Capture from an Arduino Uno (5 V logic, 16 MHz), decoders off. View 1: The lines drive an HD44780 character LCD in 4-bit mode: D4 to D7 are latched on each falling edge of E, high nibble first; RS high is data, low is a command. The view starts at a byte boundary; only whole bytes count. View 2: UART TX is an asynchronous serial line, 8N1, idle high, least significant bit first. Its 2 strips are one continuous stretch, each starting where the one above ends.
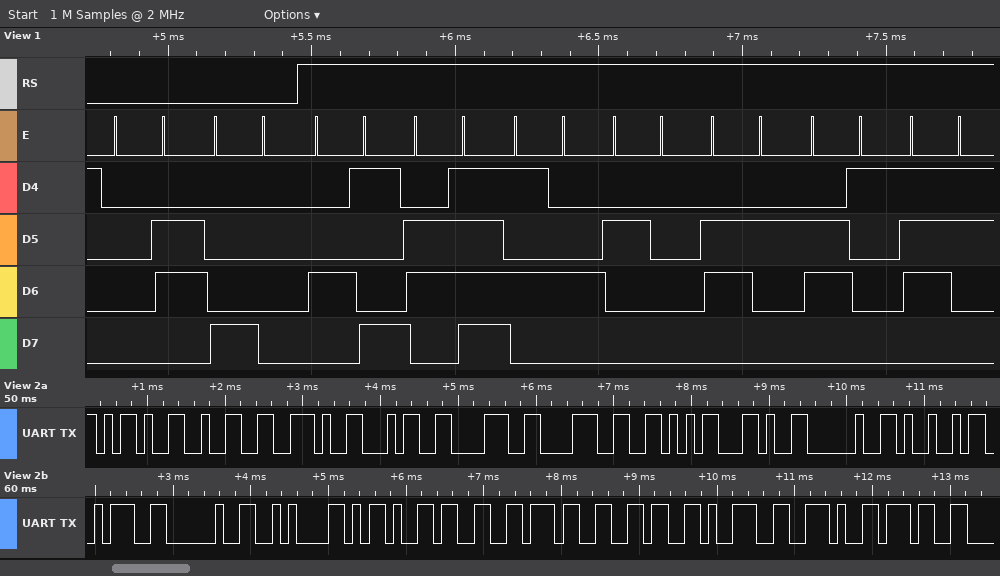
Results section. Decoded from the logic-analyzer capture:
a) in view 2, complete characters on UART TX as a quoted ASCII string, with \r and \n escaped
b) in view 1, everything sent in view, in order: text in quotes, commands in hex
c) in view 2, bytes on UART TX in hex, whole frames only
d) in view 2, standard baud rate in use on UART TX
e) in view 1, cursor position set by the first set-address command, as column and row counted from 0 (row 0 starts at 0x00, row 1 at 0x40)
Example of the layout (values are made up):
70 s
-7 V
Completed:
"-2.488V, I: \n-3769.7"
0x06 0x80 "IoT bas"
2D 32 2E 34 38 38 56 2C 20 49 3A 20 0A 2D 33 37 36 39 2E 37
9600 baud
column 0, row 0
